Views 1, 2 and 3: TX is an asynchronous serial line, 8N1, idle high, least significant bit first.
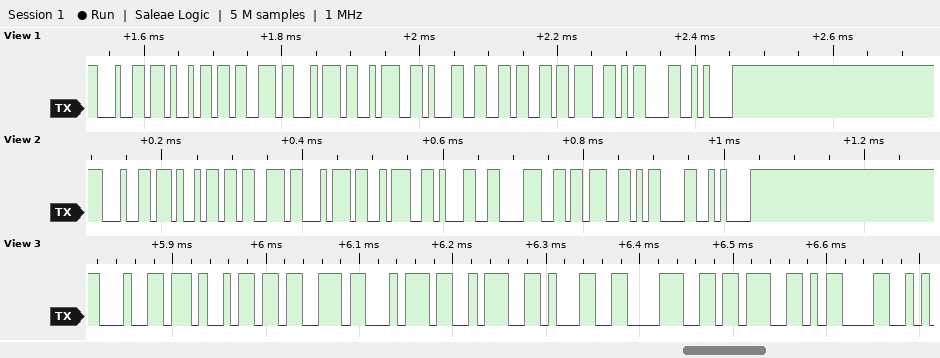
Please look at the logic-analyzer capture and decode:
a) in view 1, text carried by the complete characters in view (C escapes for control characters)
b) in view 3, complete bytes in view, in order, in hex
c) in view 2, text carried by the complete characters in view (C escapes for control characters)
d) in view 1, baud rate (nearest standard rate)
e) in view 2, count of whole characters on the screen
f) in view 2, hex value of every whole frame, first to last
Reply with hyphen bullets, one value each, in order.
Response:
- "dist:16;\r\n"
- 64 69 73 74 3A 31 38 3B 0D
- "dist:18;\r\n"
- 115200 baud
- 10
- 64 69 73 74 3A 31 38 3B 0D 0A
